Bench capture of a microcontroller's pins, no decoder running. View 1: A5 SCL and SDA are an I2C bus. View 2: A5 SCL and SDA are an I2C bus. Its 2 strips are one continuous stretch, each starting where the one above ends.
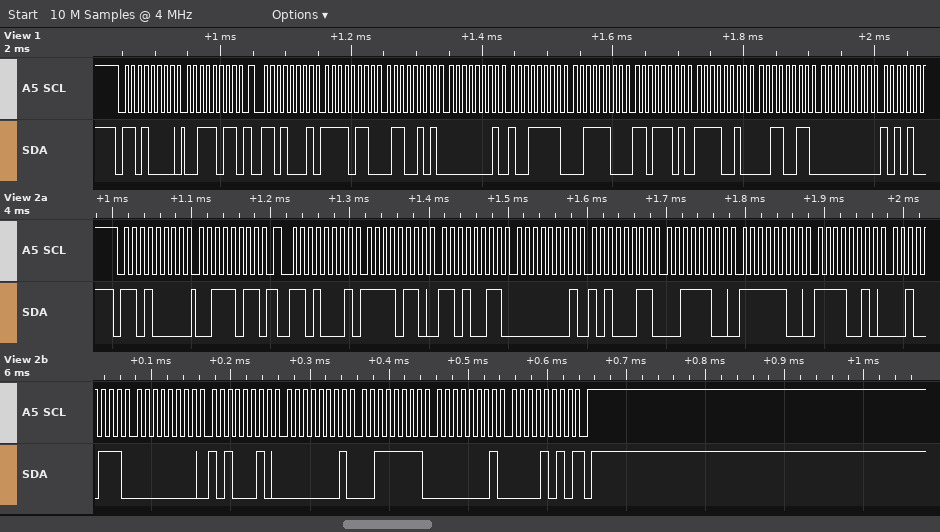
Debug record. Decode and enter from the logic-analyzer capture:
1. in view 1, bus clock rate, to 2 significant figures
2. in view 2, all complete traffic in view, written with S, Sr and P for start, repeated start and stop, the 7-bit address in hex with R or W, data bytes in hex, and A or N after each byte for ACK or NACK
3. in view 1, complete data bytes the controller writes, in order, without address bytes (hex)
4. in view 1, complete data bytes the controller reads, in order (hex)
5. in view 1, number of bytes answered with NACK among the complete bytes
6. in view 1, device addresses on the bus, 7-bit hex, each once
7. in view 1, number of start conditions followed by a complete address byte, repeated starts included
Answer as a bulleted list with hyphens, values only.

- 100 kHz
- S 68W A 3B A Sr 68R A F6 A D3 A 01 A A3 A 3C A FC A F2 A 27 A 00 A A2 A 01 A 3F A 01 A 0A N P
- 3B
- F6 65 01 9F 3C DD F2 33 00
- 0
- 0x68
- 2
